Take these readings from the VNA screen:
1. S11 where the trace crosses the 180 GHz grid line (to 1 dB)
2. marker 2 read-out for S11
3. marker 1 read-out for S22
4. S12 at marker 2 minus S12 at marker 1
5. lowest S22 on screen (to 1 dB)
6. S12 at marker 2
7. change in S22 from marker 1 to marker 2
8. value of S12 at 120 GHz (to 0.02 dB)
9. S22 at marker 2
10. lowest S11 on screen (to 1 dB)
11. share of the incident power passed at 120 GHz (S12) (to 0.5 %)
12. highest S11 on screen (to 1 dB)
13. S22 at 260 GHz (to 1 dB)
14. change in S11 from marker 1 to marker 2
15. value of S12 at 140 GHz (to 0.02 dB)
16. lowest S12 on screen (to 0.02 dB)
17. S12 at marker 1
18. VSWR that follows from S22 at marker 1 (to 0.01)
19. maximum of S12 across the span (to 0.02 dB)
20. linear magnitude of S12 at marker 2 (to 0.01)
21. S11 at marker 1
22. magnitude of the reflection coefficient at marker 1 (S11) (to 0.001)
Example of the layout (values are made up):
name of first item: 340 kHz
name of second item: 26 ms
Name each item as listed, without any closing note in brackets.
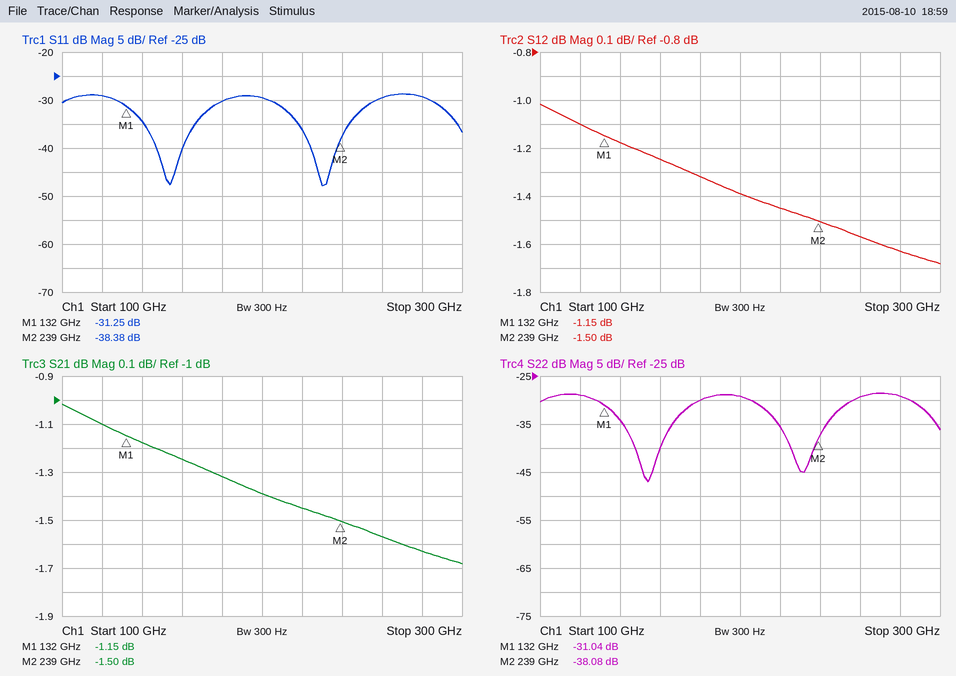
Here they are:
S11 where the trace crosses the 180 GHz grid line: -30 dB
marker 2 read-out for S11: -38.38 dB
marker 1 read-out for S22: -31.04 dB
S12 at marker 2 minus S12 at marker 1: -0.35 dB
lowest S22 on screen: -47 dB
S12 at marker 2: -1.50 dB
change in S22 from marker 1 to marker 2: -7.04 dB
value of S12 at 120 GHz: -1.10 dB
S22 at marker 2: -38.08 dB
lowest S11 on screen: -48 dB
share of the incident power passed at 120 GHz (S12): 77.5 %
highest S11 on screen: -29 dB
S22 at 260 GHz: -29 dB
change in S11 from marker 1 to marker 2: -7.13 dB
value of S12 at 140 GHz: -1.18 dB
lowest S12 on screen: -1.68 dB
S12 at marker 1: -1.15 dB
VSWR that follows from S22 at marker 1: 1.06
maximum of S12 across the span: -1.02 dB
linear magnitude of S12 at marker 2: 0.84
S11 at marker 1: -31.25 dB
magnitude of the reflection coefficient at marker 1 (S11): 0.027
